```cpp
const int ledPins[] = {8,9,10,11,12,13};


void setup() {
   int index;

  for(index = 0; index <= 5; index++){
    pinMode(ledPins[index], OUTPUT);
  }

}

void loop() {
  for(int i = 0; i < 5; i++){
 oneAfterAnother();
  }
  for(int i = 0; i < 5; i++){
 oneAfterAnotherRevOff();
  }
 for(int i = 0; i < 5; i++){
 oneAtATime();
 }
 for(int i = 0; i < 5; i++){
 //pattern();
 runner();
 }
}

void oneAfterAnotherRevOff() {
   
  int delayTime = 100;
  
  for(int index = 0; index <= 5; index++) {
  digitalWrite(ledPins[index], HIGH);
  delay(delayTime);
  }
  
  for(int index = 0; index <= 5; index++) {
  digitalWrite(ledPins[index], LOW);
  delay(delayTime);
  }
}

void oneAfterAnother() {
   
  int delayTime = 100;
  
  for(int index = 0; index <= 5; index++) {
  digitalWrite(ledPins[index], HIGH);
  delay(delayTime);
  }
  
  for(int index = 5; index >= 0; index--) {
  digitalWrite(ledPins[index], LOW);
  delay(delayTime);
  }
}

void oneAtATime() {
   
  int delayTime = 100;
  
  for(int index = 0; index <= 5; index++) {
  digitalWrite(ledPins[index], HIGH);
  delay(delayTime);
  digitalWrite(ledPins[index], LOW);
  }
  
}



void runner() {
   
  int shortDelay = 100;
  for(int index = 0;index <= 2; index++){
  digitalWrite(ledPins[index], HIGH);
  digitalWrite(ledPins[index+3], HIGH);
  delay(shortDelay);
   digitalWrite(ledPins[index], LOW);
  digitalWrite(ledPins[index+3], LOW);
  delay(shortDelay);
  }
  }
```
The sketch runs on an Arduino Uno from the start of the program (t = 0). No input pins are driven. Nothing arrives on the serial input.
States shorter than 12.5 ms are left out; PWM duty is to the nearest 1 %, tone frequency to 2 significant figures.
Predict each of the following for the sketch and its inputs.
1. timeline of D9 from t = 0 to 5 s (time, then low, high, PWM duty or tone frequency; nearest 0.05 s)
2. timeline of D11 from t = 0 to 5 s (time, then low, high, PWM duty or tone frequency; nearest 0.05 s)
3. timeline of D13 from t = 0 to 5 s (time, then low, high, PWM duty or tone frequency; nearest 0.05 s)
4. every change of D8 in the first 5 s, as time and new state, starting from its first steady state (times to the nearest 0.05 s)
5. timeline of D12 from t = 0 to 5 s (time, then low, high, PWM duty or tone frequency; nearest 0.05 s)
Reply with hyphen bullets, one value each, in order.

- 0 s low; 0.1 s high; 1 s low; 1.3 s high; 2.2 s low; 2.5 s high; 3.4 s low; 3.7 s high; 4.6 s low; 4.9 s high
- 0 s low; 0.3 s high; 0.8 s low; 1.5 s high; 2 s low; 2.7 s high; 3.2 s low; 3.9 s high; 4.4 s low
- 0 s low; 0.5 s high; 0.6 s low; 1.7 s high; 1.8 s low; 2.9 s high; 3 s low; 4.1 s high; 4.2 s low
- 0 s high; 1.1 s low; 1.2 s high; 2.3 s low; 2.4 s high; 3.5 s low; 3.6 s high; 4.7 s low; 4.8 s high
- 0 s low; 0.4 s high; 0.7 s low; 1.6 s high; 1.9 s low; 2.8 s high; 3.1 s low; 4 s high; 4.3 s low
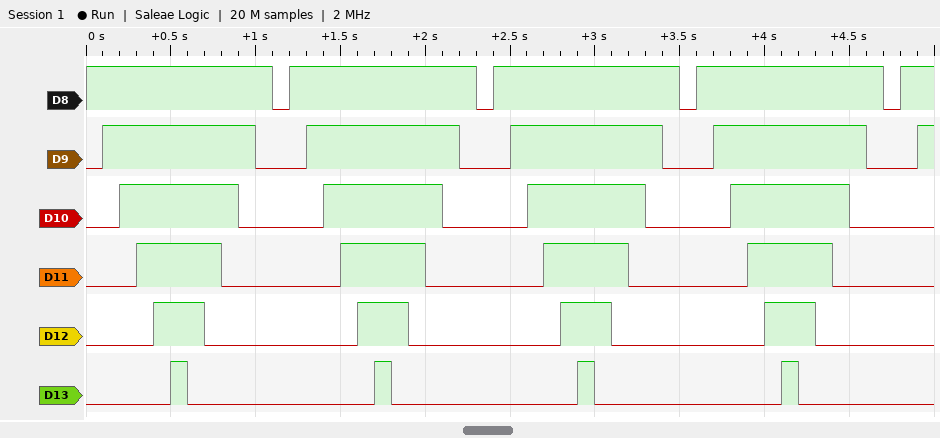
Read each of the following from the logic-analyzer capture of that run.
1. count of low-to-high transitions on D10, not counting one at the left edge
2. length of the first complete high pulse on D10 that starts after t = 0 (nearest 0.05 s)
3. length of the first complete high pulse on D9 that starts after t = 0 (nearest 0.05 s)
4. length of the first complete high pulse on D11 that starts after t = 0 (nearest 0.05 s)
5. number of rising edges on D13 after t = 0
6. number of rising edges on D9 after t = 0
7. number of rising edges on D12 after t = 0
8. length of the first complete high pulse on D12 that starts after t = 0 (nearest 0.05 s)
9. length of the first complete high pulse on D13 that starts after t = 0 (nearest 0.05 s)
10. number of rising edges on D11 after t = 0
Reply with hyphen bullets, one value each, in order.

- 4
- 0.70 s
- 0.90 s
- 0.50 s
- 4
- 5
- 4
- 0.30 s
- 0.10 s
- 4
